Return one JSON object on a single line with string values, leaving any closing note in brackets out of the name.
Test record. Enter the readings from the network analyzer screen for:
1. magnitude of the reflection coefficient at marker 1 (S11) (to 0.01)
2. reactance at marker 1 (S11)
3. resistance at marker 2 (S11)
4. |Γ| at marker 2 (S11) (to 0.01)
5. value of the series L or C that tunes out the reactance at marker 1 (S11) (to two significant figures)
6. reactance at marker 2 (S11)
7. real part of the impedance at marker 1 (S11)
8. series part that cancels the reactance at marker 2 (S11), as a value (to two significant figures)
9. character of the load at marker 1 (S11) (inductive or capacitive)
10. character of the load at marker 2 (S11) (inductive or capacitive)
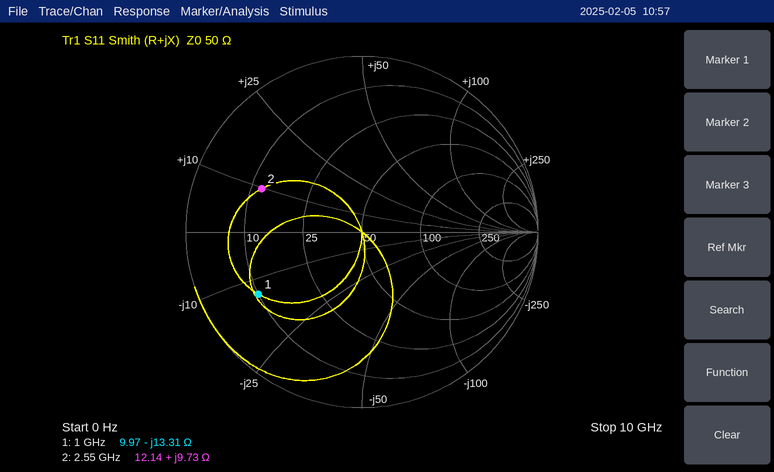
{"magnitude of the reflection coefficient at marker 1 (S11)": "0.69", "reactance at marker 1": "-13.31 Ω", "resistance at marker 2": "12.14 Ω", "|Γ| at marker 2 (S11)": "0.62", "value of the series L or C that tunes out the reactance at marker 1 (S11)": "2.1 nH", "reactance at marker 2": "+9.73 Ω", "real part of the impedance at marker 1": "9.97 Ω", "series part that cancels the reactance at marker 2 (S11), as a value": "6.4 pF", "character of the load at marker 1 (S11)": "capacitive", "character of the load at marker 2 (S11)": "inductive"}
